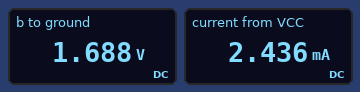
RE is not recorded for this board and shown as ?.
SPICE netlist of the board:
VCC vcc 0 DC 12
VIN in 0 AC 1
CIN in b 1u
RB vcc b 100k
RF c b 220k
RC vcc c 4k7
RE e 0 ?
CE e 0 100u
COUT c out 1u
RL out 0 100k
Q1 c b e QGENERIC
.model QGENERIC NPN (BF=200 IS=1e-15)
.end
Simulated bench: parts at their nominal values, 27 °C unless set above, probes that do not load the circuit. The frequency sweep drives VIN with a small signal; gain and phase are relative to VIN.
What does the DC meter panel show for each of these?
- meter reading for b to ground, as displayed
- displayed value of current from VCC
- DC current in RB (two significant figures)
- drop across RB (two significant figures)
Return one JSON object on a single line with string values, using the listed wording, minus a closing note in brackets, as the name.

{"meter reading for b to ground, as displayed": "1.688 V", "displayed value of current from VCC": "2.436 mA", "DC current in RB": "100 µA", "drop across RB": "10 V"}
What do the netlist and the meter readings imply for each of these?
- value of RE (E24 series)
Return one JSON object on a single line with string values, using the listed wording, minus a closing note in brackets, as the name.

{"value of RE": "390 Ω"}
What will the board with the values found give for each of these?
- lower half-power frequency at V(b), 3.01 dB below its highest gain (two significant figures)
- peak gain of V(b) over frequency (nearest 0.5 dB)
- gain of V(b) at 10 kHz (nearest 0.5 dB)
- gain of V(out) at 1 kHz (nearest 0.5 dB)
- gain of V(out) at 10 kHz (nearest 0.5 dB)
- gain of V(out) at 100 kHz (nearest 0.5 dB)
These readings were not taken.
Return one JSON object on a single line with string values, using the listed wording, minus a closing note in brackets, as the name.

{"lower half-power frequency at V(b), 3.01 dB below its highest gain": "7.7 kHz", "peak gain of V(b) over frequency": "0 dB", "gain of V(b) at 10 kHz": "-2.0 dB", "gain of V(out) at 1 kHz": "4.5 dB", "gain of V(out) at 10 kHz": "20.0 dB", "gain of V(out) at 100 kHz": "22.0 dB"}
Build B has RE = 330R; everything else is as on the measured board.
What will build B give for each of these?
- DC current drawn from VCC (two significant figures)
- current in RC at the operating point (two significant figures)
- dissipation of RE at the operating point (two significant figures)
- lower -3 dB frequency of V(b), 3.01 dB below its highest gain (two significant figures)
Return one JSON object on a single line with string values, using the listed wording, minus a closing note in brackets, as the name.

{"DC current drawn from VCC": "2.5 mA", "current in RC at the operating point": "2.4 mA", "dissipation of RE at the operating point": "2.0 mW", "lower -3 dB frequency of V(b), 3.01 dB below its highest gain": "7.8 kHz"}
